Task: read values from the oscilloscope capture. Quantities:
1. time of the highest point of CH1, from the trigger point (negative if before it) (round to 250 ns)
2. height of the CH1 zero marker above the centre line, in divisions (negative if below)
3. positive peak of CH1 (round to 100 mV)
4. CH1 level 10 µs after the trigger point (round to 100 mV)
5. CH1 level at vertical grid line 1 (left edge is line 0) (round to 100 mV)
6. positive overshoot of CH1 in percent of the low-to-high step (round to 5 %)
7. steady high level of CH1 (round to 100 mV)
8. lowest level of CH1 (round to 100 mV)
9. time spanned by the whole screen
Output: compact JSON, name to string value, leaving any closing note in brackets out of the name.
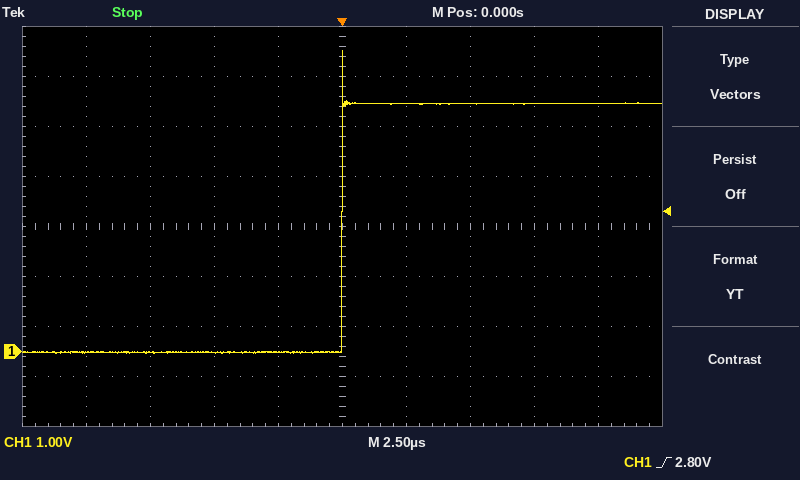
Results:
{"time of the highest point of CH1, from the trigger point (negative if before it)": "0.00 µs", "height of the CH1 zero marker above the centre line, in divisions": "-2.5 div", "positive peak of CH1": "6.0 V", "CH1 level 10 µs after the trigger point": "5.0 V", "CH1 level at vertical grid line 1 (left edge is line 0)": "0.0 V", "positive overshoot of CH1 in percent of the low-to-high step": "20 %", "steady high level of CH1": "5.0 V", "lowest level of CH1": "0.0 V", "time spanned by the whole screen": "25 µs"}
